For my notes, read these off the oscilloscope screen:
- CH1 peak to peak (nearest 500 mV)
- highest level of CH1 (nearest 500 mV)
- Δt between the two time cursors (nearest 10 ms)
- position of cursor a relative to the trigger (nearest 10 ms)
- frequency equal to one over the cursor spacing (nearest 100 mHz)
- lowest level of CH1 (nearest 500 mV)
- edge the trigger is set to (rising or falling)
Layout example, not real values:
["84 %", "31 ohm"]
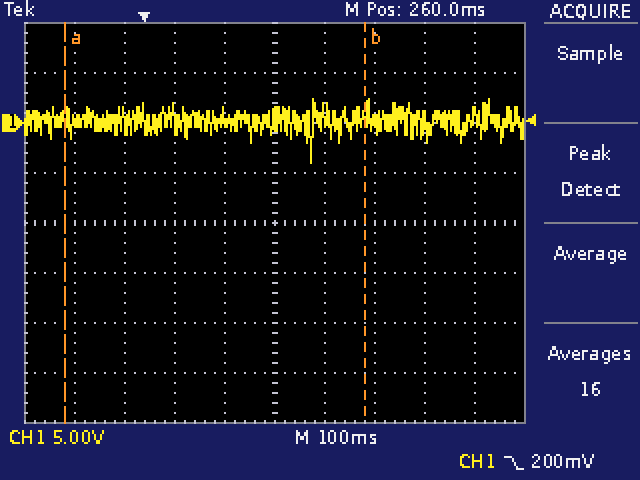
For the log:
["6.5 V", "2.5 V", "600 ms", "-160 ms", "1.7 Hz", "-4.0 V", "falling"]
